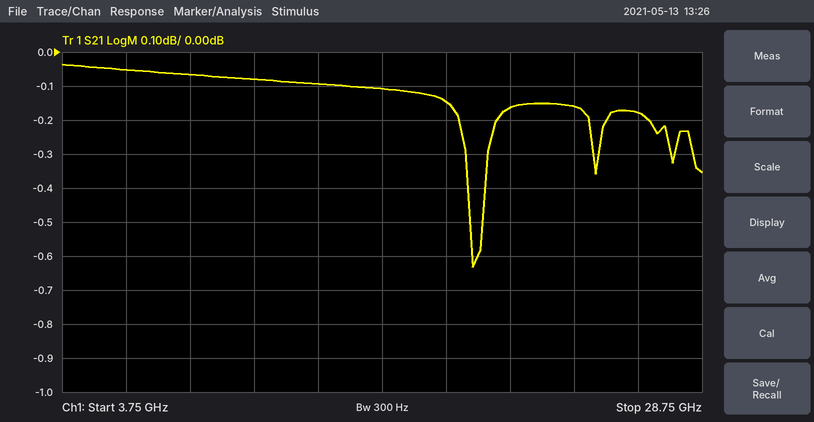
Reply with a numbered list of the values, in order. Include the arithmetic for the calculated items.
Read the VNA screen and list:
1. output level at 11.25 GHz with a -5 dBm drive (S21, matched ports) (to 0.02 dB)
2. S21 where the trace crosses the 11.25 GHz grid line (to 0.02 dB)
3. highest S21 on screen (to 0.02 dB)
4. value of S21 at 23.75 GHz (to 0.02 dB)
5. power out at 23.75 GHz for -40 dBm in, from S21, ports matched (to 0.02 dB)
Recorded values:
1. -5 dBm + (-0.08 dB) = -5.08 dBm
2. -0.08 dB
3. -0.04 dB
4. -0.16 dB
5. -40 dBm + (-0.16 dB) = -40.16 dBm
